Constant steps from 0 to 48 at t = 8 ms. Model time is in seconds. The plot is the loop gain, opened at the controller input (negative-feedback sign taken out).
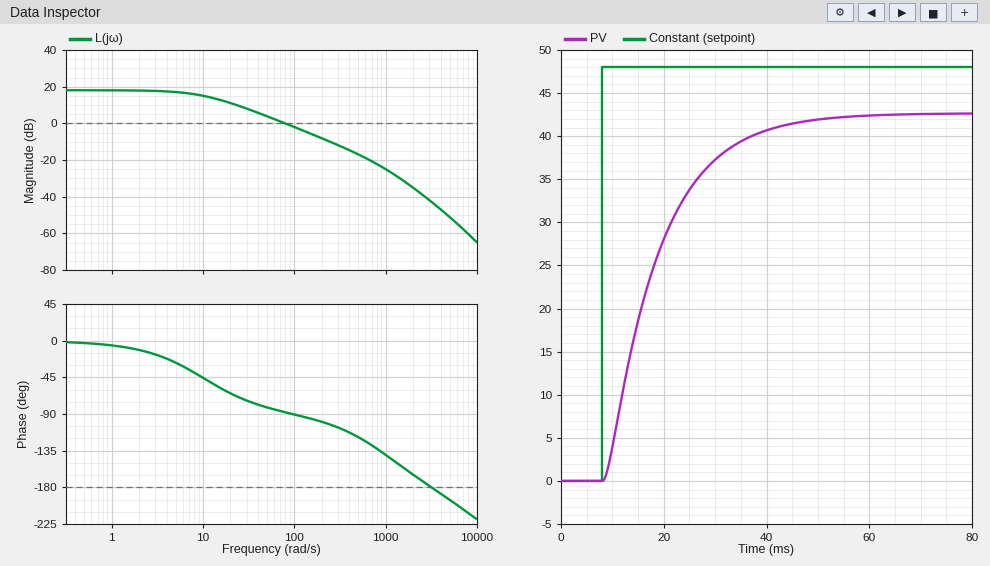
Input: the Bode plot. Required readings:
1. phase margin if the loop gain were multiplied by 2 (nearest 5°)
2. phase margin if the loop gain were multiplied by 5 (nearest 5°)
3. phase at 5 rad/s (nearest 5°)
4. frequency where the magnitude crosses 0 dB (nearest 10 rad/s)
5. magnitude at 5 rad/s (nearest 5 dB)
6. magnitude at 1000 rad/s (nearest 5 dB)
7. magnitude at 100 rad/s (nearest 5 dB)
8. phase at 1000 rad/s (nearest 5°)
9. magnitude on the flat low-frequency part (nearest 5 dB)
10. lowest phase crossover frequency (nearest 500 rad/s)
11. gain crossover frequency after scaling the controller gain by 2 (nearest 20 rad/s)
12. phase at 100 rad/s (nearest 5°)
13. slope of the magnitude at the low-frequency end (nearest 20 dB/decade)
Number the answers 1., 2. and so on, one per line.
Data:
1. 85°
2. 70°
3. -25°
4. 80 rad/s
5. 15 dB
6. -25 dB
7. 0 dB
8. -140°
9. 20 dB
10. 3000 rad/s
11. 160 rad/s
12. -90°
13. 0 dB/decade
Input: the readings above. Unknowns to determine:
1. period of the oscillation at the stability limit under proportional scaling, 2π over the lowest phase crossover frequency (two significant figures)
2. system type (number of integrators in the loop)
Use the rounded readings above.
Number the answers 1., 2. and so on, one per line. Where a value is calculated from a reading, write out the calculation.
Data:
1. 2π / 3000 = 0.0021 s
2. 0
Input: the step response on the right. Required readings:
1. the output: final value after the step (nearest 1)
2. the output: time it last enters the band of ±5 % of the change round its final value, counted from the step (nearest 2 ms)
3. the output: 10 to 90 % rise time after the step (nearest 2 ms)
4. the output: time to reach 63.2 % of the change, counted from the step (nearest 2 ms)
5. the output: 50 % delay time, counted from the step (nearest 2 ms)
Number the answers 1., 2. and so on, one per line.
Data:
1. 43
2. 32 ms
3. 22 ms
4. 12 ms
5. 8 ms
